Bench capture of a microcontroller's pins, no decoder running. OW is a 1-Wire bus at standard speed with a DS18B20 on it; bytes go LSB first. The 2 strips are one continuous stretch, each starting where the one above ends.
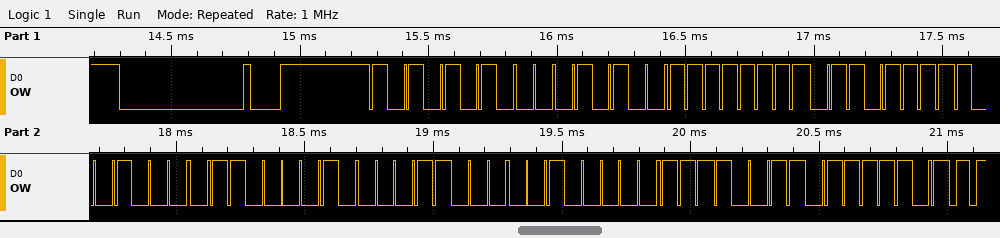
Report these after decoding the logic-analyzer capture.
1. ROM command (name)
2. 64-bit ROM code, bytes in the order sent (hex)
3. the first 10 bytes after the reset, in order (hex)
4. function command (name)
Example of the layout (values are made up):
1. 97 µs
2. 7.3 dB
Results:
1. Match ROM
2. 28 FF F6 09 43 18 04 CF
3. 55 28 FF F6 09 43 18 04 CF BE
4. Read Scratchpad
